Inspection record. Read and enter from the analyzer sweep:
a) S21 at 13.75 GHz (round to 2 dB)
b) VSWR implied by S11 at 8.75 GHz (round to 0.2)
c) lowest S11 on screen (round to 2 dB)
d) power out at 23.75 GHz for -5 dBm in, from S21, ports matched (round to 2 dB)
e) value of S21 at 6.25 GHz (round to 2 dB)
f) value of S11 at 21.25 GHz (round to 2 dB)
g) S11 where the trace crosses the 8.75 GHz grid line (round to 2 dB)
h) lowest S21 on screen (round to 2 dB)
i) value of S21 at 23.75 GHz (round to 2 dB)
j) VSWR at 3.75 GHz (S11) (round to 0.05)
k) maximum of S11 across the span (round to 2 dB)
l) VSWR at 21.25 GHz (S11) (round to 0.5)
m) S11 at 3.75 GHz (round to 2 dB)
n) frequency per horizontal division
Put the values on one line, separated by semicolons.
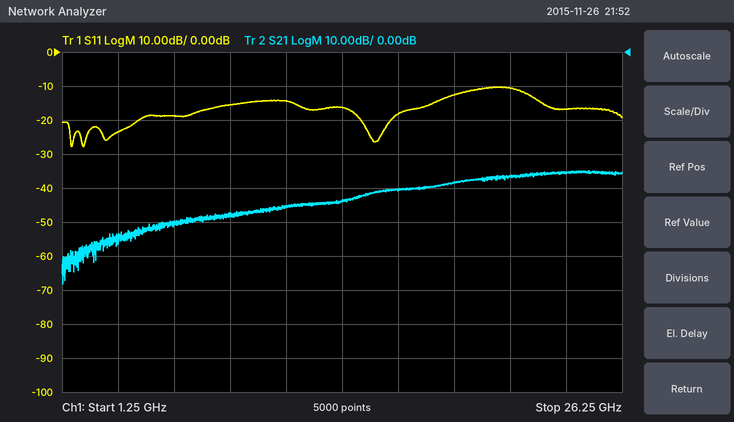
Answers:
-44 dB; 1.4; -28 dB; -40 dBm; -50 dB; -10 dB; -16 dB; -68 dB; -36 dB; 1.15; -10 dB; 2.0; -24 dB; 2.5 GHz
